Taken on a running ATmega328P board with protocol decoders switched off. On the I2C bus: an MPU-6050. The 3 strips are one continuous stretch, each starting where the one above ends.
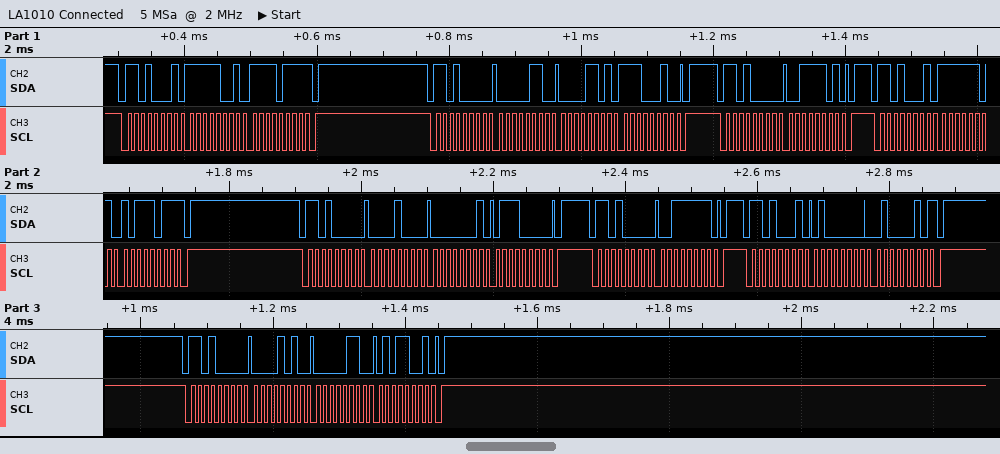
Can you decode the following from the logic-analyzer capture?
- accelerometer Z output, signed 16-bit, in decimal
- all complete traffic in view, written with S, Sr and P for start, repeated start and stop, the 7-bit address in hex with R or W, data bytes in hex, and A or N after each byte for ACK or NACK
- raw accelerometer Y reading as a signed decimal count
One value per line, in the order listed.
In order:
16450
S 68R A F9 A F7 N P S 68W A 06 A 0D A E2 A P S 68W A 3D A P S 68R A FD A BB N P S 68W A 08 A 01 A 70 A P S 68W A 3F A P S 68R A 40 A 42 N P S 68W A 0A A 06 A 59 A P
-581
